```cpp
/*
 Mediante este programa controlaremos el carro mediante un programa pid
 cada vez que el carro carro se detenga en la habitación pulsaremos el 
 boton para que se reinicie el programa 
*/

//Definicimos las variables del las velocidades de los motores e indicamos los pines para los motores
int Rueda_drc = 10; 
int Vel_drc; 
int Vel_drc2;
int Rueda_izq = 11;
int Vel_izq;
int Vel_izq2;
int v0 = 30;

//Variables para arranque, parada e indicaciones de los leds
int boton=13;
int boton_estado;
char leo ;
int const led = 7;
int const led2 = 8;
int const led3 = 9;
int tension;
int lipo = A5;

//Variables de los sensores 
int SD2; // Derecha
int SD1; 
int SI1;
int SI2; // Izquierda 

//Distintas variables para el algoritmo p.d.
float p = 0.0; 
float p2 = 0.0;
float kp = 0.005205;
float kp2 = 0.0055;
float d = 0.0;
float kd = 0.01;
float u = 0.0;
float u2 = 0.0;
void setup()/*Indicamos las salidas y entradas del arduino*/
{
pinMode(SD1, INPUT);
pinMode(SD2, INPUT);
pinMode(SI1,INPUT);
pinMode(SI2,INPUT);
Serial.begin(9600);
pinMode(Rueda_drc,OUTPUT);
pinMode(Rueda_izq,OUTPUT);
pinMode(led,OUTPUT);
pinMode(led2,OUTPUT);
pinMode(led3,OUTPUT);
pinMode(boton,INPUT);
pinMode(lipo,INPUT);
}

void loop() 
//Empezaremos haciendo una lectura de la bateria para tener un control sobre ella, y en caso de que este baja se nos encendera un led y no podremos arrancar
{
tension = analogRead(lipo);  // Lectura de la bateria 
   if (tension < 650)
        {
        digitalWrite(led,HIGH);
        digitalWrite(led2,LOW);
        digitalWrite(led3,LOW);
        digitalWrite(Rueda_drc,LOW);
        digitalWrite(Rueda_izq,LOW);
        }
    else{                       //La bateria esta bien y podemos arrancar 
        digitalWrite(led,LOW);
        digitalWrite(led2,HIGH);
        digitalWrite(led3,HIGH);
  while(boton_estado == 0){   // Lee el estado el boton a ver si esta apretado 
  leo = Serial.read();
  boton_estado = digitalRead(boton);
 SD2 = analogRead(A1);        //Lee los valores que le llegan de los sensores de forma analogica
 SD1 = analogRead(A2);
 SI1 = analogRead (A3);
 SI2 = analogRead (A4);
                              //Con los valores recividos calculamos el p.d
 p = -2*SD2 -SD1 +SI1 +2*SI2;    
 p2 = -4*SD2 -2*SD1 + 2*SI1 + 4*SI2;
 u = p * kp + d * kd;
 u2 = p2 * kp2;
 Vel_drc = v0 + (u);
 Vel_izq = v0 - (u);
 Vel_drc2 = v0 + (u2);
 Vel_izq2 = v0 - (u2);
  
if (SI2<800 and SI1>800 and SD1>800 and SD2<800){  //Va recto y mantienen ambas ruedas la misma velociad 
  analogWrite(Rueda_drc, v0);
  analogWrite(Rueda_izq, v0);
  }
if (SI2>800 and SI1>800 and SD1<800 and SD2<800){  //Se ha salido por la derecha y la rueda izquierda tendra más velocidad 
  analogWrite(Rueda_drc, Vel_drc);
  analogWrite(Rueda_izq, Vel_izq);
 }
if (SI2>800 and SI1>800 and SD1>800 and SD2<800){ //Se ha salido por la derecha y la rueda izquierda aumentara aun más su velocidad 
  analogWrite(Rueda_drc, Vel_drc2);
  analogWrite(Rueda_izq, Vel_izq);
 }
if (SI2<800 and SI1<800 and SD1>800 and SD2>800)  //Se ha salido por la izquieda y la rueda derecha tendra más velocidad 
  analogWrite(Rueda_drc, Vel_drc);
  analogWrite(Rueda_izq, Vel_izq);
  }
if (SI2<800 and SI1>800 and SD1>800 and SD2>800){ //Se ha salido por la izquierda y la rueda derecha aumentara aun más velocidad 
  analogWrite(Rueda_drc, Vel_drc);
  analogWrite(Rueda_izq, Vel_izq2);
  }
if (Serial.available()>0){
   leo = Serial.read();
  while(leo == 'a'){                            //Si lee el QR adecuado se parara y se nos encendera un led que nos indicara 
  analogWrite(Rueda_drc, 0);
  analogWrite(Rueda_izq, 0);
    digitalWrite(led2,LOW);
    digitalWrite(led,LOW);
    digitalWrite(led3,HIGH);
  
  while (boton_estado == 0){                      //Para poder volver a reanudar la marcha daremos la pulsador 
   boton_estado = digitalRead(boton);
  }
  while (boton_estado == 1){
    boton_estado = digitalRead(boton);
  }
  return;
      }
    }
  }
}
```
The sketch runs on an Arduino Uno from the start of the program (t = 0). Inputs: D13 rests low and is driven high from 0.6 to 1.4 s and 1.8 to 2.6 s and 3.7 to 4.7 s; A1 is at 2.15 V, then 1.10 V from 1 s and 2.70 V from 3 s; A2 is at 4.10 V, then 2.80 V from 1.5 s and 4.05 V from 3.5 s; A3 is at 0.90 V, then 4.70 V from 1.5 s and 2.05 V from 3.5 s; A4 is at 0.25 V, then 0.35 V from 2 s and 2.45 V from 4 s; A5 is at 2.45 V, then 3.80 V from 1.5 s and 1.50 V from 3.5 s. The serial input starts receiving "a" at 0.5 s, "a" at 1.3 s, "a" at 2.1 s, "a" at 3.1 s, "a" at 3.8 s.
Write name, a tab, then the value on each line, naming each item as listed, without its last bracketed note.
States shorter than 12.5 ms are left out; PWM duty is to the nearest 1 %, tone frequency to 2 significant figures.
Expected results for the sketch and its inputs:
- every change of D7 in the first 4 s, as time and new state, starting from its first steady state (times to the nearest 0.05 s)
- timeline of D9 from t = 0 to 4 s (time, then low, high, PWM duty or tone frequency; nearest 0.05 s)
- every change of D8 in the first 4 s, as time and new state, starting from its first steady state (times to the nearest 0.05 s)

every change of D7 in the first 4 s, as time and new state, starting from its first steady state	0 s high; 1.5 s low; 3.7 s high
timeline of D9 from t = 0 to 4 s	0 s low; 1.5 s high; 3.7 s low
every change of D8 in the first 4 s, as time and new state, starting from its first steady state	0 s low; 1.5 s high; 2.1 s low; 2.6 s high; 3.7 s low
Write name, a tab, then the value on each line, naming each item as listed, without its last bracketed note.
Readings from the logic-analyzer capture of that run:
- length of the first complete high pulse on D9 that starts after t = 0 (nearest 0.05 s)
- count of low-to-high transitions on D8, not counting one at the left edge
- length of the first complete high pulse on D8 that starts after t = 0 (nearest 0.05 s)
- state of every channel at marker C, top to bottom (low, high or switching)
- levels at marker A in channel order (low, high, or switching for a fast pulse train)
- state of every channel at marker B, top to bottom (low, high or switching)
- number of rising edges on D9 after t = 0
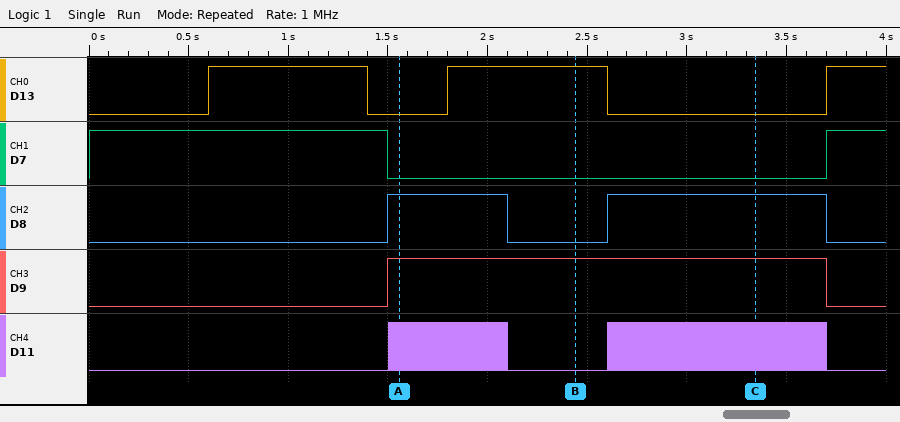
length of the first complete high pulse on D9 that starts after t = 0	2.20 s
count of low-to-high transitions on D8, not counting one at the left edge	2
length of the first complete high pulse on D8 that starts after t = 0	0.60 s
state of every channel at marker C, top to bottom	D13 low, D7 low, D8 high, D9 high, D11 switching
levels at marker A in channel order	D13 low, D7 low, D8 high, D9 high, D11 switching
state of every channel at marker B, top to bottom	D13 high, D7 low, D8 low, D9 high, D11 low
number of rising edges on D9 after t = 0	1
